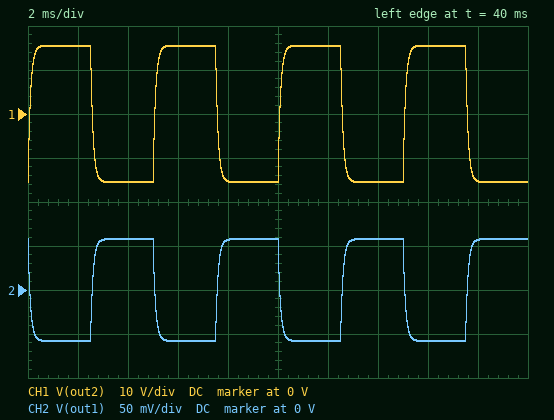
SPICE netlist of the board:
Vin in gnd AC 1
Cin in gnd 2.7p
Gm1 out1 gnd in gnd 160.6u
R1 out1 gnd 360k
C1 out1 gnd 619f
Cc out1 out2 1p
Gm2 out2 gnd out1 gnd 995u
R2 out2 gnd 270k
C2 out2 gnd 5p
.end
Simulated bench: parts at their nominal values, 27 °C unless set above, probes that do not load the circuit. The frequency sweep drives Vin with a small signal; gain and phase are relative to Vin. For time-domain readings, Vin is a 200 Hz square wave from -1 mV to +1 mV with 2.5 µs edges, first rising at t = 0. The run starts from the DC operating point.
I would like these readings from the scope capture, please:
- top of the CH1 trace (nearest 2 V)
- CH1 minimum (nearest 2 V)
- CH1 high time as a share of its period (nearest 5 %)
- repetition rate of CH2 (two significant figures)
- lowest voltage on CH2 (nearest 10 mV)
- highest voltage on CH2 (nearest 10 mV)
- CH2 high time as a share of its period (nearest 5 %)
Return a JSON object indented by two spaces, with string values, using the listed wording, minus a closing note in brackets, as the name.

{
  "top of the CH1 trace": "16 V",
  "CH1 minimum": "-16 V",
  "CH1 high time as a share of its period": "50 %",
  "repetition rate of CH2": "200 Hz",
  "lowest voltage on CH2": "-60 mV",
  "highest voltage on CH2": "60 mV",
  "CH2 high time as a share of its period": "50 %"
}
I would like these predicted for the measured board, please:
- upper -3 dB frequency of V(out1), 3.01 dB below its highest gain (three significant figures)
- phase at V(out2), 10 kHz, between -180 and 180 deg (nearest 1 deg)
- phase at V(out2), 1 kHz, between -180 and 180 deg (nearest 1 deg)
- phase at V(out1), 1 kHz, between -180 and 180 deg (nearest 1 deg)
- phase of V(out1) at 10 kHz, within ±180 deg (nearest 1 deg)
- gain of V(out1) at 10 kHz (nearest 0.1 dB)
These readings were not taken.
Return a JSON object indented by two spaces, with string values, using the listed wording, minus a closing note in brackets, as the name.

{
  "upper -3 dB frequency of V(out1), 3.01 dB below its highest gain": "1.61 kHz",
  "phase at V(out2), 10 kHz, between -180 and 180 deg": "-81 deg",
  "phase at V(out2), 1 kHz, between -180 and 180 deg": "-32 deg",
  "phase at V(out1), 1 kHz, between -180 and 180 deg": "149 deg",
  "phase of V(out1) at 10 kHz, within ±180 deg": "105 deg",
  "gain of V(out1) at 10 kHz": "19.3 dB"
}
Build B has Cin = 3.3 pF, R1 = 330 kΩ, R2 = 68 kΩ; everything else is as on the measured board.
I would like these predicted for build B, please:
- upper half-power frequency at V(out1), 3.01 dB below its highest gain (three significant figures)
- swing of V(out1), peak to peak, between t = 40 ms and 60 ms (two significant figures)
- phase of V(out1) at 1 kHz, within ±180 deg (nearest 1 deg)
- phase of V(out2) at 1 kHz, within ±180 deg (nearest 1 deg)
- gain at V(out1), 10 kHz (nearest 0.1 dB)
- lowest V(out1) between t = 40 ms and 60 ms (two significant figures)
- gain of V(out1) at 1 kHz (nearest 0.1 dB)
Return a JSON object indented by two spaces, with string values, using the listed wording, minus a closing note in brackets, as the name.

{
  "upper half-power frequency at V(out1), 3.01 dB below its highest gain": "6.84 kHz",
  "swing of V(out1), peak to peak, between t = 40 ms and 60 ms": "110 mV",
  "phase of V(out1) at 1 kHz, within ±180 deg": "172 deg",
  "phase of V(out2) at 1 kHz, within ±180 deg": "-8 deg",
  "gain at V(out1), 10 kHz": "29.5 dB",
  "lowest V(out1) between t = 40 ms and 60 ms": "-53 mV",
  "gain of V(out1) at 1 kHz": "34.4 dB"
}
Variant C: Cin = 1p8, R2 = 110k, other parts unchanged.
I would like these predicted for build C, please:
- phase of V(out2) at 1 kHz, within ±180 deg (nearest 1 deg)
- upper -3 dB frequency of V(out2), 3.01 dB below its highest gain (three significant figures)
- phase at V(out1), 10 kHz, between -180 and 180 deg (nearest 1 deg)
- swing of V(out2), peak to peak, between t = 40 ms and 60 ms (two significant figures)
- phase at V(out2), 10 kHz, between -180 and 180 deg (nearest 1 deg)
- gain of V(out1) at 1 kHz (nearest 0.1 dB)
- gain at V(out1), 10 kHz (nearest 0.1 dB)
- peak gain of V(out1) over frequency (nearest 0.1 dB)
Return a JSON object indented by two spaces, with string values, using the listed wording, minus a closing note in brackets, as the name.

{
  "phase of V(out2) at 1 kHz, within ±180 deg": "-14 deg",
  "upper -3 dB frequency of V(out2), 3.01 dB below its highest gain": "3.92 kHz",
  "phase at V(out1), 10 kHz, between -180 and 180 deg": "114 deg",
  "swing of V(out2), peak to peak, between t = 40 ms and 60 ms": "13 V",
  "phase at V(out2), 10 kHz, between -180 and 180 deg": "-69 deg",
  "gain of V(out1) at 1 kHz": "35.0 dB",
  "gain at V(out1), 10 kHz": "26.5 dB",
  "peak gain of V(out1) over frequency": "35.2 dB"
}
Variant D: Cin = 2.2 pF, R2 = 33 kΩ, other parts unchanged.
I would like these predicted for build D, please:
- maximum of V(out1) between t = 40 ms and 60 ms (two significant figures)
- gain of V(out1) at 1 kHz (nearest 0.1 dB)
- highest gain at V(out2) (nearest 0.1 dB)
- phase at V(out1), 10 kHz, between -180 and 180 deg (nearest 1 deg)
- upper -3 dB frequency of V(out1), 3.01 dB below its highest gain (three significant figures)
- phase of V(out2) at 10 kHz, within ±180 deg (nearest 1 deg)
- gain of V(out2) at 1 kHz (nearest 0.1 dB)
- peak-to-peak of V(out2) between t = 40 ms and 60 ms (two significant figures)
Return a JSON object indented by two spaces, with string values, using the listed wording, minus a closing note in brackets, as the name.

{
  "maximum of V(out1) between t = 40 ms and 60 ms": "58 mV",
  "gain of V(out1) at 1 kHz": "35.2 dB",
  "highest gain at V(out2)": "65.6 dB",
  "phase at V(out1), 10 kHz, between -180 and 180 deg": "142 deg",
  "upper -3 dB frequency of V(out1), 3.01 dB below its highest gain": "12.6 kHz",
  "phase of V(out2) at 10 kHz, within ±180 deg": "-38 deg",
  "gain of V(out2) at 1 kHz": "65.5 dB",
  "peak-to-peak of V(out2) between t = 40 ms and 60 ms": "3.8 V"
}
